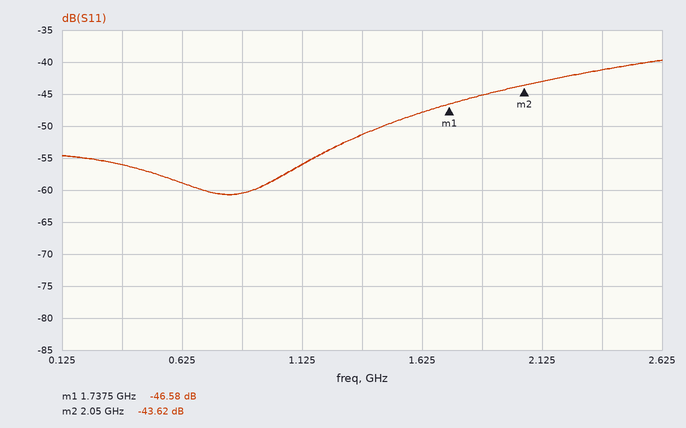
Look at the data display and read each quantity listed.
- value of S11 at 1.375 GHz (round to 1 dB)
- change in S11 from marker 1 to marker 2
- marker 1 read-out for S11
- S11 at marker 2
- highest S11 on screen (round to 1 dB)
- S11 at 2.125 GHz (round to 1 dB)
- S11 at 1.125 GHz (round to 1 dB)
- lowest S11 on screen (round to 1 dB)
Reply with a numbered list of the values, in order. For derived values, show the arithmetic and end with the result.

1. -51 dB
2. -43.62 − (-46.58) = 2.96 dB
3. -46.58 dB
4. -43.62 dB
5. -40 dB
6. -43 dB
7. -56 dB
8. -61 dB
